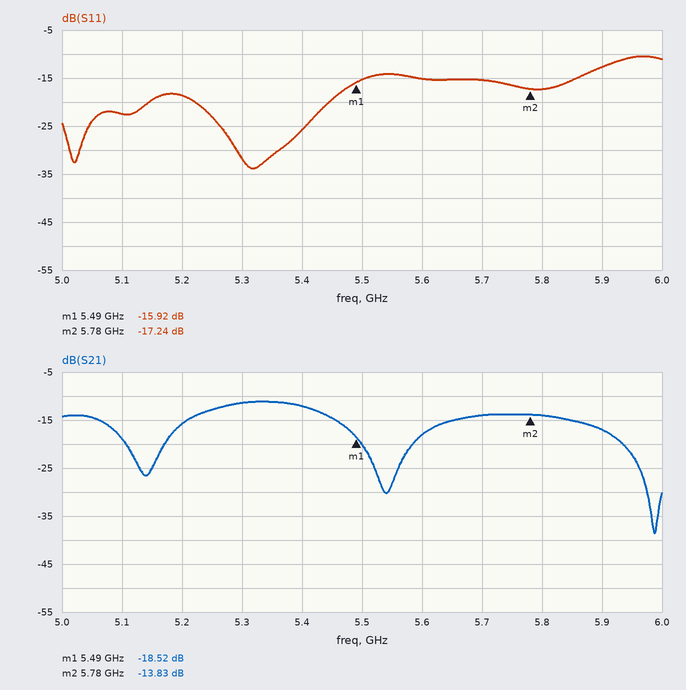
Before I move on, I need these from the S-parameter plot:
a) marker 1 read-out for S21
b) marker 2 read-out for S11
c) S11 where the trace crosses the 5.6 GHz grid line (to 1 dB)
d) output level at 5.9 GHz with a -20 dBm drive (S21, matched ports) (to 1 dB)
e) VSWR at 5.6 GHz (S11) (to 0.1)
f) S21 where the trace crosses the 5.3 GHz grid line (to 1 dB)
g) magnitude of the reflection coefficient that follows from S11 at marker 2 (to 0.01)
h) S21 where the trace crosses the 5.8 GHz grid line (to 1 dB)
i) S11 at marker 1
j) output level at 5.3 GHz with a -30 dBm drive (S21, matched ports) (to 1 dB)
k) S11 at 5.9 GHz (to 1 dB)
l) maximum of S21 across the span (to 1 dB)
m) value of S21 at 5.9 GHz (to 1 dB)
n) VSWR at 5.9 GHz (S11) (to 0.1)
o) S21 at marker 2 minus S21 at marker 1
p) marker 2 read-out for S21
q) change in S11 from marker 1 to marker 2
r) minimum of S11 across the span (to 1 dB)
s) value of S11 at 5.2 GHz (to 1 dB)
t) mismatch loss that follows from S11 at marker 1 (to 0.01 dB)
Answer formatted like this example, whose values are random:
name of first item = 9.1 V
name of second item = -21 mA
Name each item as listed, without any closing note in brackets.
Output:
marker 1 read-out for S21 = -18.52 dB
marker 2 read-out for S11 = -17.24 dB
S11 where the trace crosses the 5.6 GHz grid line = -15 dB
output level at 5.9 GHz with a -20 dBm drive (S21, matched ports) = -37 dBm
VSWR at 5.6 GHz (S11) = 1.4
S21 where the trace crosses the 5.3 GHz grid line = -11 dB
magnitude of the reflection coefficient that follows from S11 at marker 2 = 0.14
S21 where the trace crosses the 5.8 GHz grid line = -14 dB
S11 at marker 1 = -15.92 dB
output level at 5.3 GHz with a -30 dBm drive (S21, matched ports) = -41 dBm
S11 at 5.9 GHz = -13 dB
maximum of S21 across the span = -11 dB
value of S21 at 5.9 GHz = -17 dB
VSWR at 5.9 GHz (S11) = 1.6
S21 at marker 2 minus S21 at marker 1 = 4.69 dB
marker 2 read-out for S21 = -13.83 dB
change in S11 from marker 1 to marker 2 = -1.32 dB
minimum of S11 across the span = -34 dB
value of S11 at 5.2 GHz = -19 dB
mismatch loss that follows from S11 at marker 1 = 0.11 dB
